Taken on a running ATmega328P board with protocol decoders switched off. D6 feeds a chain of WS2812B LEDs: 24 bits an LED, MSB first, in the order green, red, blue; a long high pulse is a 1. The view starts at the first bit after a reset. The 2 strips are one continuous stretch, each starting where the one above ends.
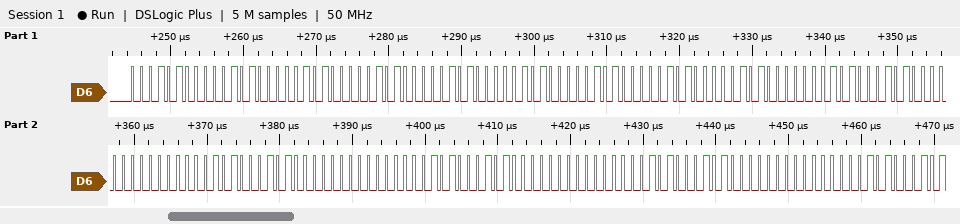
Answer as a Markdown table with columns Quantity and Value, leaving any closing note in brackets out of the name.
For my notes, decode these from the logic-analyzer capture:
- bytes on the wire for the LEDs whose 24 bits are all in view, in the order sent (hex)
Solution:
| Quantity | Value |
|---|---|
| bytes on the wire for the LEDs whose 24 bits are all in view, in the order sent | 14 14 14 14 14 14 14 14 14 05 14 00 05 14 00 05 14 00 05 14 00 |
